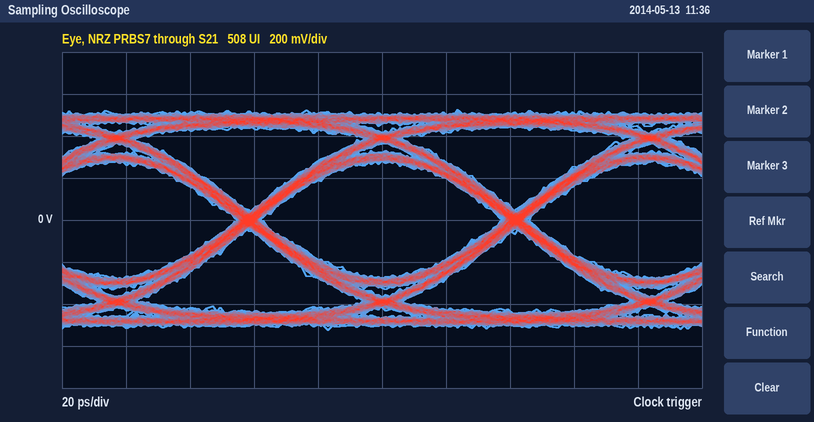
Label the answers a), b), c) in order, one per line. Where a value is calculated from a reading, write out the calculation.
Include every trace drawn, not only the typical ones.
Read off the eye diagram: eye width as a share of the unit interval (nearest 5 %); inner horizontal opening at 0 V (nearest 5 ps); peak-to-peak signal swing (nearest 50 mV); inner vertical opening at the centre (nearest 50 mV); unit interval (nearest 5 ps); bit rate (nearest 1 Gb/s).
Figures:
a) 75 ps / 85 ps ≈ 88.2 %, so 90 % to the nearest 5 %
b) 75 ps
c) 1.05 V
d) 550 mV
e) 85 ps
f) 12 Gb/s
